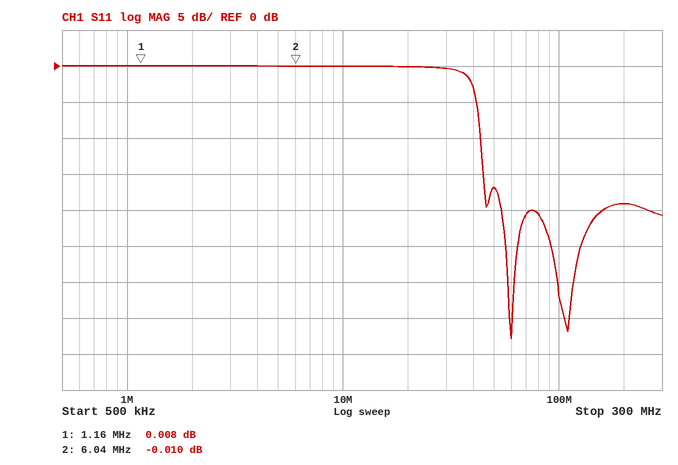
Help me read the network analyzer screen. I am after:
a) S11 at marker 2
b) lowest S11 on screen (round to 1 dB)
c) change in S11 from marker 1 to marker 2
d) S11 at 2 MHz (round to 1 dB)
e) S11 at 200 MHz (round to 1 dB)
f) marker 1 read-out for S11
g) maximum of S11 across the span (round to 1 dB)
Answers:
-0.010 dB
-38 dB
-0.018 dB
0 dB
-19 dB
0.008 dB
0 dB
